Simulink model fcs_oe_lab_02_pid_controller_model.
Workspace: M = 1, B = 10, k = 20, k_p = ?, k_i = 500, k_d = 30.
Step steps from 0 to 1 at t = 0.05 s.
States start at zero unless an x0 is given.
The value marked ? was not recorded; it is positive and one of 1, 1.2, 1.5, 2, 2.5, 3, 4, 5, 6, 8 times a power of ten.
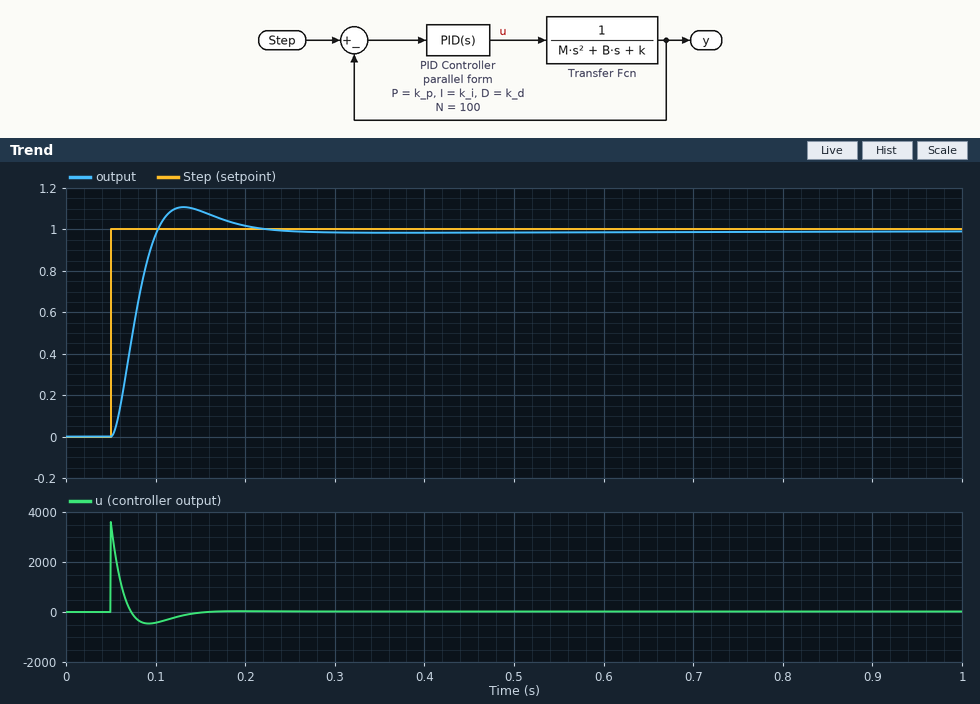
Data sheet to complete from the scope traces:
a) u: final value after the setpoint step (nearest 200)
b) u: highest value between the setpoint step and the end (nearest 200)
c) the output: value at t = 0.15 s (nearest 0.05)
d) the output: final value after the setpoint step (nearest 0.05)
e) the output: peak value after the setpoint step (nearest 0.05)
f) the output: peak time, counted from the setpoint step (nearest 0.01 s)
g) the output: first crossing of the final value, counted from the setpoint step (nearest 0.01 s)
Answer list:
0
3600
1.10
1.00
1.10
0.08 s
0.05 s
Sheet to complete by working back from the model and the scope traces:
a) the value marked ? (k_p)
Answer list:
600
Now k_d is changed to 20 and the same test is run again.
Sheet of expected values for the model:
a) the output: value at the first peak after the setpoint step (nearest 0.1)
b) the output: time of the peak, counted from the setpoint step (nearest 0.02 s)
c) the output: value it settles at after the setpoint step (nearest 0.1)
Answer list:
1.2
0.10 s
1.0
